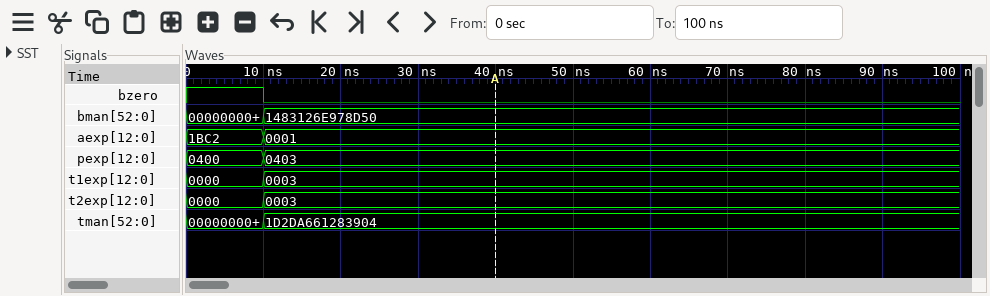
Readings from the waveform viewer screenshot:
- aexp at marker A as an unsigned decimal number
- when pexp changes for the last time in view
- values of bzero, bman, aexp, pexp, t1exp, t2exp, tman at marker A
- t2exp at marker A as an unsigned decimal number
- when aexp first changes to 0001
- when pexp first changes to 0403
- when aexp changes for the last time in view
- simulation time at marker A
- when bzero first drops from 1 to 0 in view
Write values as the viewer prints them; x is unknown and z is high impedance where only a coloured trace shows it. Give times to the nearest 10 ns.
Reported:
1
10 ns
bzero=0, bman=1483126E978D50, aexp=0001, pexp=0403, t1exp=0003, t2exp=0003, tman=1D2DA661283904
3
10 ns
10 ns
10 ns
40 ns
10 ns
